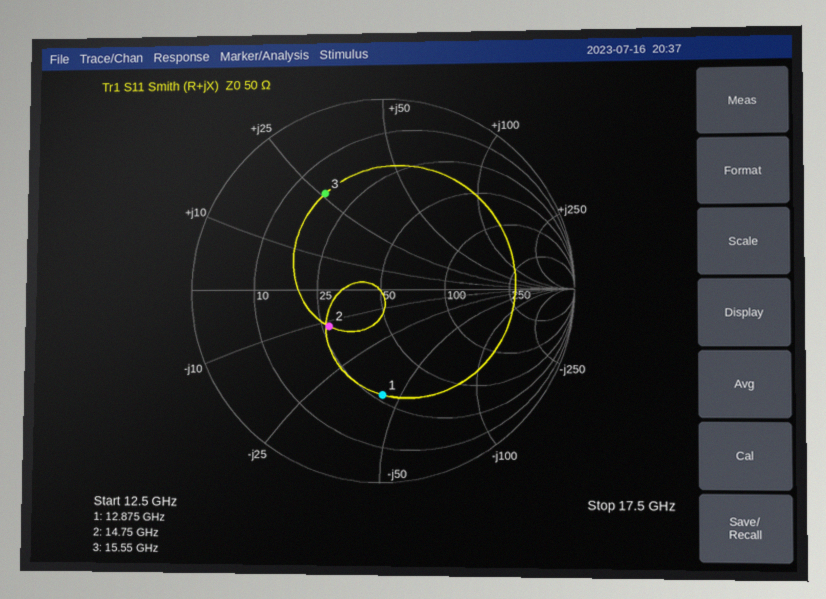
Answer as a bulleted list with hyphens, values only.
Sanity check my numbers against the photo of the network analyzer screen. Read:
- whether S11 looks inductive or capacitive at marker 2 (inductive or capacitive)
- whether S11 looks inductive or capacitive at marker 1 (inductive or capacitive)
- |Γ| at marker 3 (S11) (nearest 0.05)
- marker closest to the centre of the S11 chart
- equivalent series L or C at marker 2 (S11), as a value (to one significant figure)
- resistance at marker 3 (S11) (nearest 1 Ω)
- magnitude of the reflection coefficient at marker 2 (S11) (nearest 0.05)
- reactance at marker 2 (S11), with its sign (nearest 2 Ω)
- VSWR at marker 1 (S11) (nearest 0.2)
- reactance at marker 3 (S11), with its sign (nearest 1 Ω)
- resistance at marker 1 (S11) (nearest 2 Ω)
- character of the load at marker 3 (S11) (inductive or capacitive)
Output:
- capacitive
- capacitive
- 0.60
- marker 2
- 900 fF
- 17 Ω
- 0.35
- -12 Ω
- 3.4
- +26 Ω
- 28 Ω
- inductive
